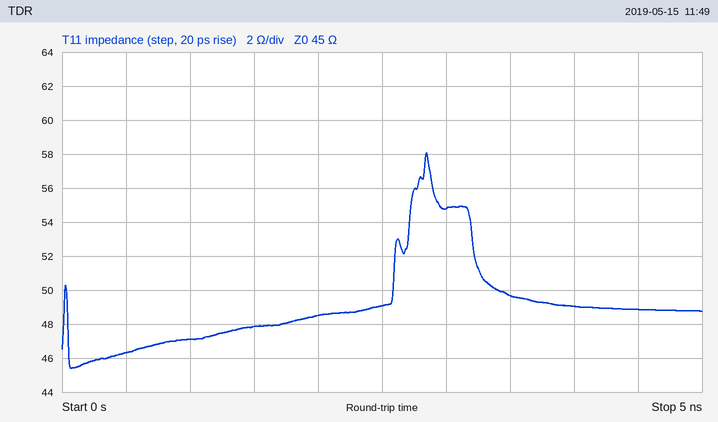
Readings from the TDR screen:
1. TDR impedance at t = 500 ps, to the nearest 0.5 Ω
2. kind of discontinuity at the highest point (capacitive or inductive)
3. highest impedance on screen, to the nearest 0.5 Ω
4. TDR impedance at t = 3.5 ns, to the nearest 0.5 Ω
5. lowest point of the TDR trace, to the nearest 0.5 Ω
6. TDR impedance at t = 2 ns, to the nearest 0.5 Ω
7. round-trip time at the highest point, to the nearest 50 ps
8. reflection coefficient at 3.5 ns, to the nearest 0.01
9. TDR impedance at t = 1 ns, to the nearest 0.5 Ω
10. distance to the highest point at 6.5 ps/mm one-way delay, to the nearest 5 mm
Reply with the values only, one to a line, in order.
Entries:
46.5 Ω
inductive
58.0 Ω
49.5 Ω
45.5 Ω
48.5 Ω
2.85 ns
+0.05
47.0 Ω
220 mm
